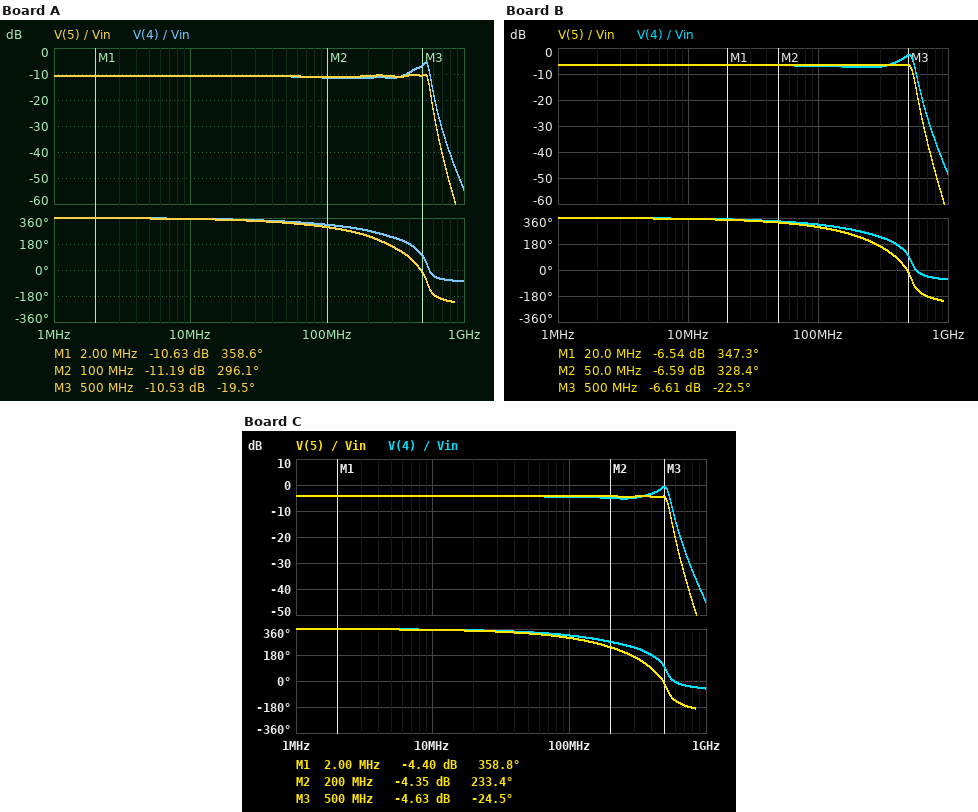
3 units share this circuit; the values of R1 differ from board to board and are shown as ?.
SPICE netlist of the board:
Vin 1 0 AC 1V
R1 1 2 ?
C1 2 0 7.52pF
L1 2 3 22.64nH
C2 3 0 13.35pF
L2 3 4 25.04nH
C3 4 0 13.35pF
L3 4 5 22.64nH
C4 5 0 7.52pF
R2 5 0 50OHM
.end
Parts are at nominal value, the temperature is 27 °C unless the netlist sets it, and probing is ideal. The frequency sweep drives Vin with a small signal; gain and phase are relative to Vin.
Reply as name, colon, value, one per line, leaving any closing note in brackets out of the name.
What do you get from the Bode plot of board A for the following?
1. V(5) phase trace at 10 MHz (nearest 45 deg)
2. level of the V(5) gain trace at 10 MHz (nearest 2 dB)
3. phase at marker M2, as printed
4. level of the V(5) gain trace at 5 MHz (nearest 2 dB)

V(5) phase trace at 10 MHz: 360 deg
level of the V(5) gain trace at 10 MHz: -10 dB
phase at marker M2, as printed: 296.1 deg
level of the V(5) gain trace at 5 MHz: -10 dB
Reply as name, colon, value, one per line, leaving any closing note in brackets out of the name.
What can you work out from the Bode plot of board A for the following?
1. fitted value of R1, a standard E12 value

fitted value of R1, a standard E12 value: 120 Ω
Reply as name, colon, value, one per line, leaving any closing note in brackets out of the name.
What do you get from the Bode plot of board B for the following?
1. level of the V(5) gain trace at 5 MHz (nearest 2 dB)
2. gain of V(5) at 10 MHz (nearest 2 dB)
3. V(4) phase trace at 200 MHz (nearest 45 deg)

level of the V(5) gain trace at 5 MHz: -6 dB
gain of V(5) at 10 MHz: -6 dB
V(4) phase trace at 200 MHz: 270 deg
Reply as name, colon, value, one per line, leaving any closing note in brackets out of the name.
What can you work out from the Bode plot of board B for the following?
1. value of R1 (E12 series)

value of R1: 56 Ω
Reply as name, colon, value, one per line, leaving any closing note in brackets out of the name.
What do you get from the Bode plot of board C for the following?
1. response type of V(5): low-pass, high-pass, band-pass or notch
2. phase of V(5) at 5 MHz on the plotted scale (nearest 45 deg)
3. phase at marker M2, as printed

response type of V(5): low-pass, high-pass, band-pass or notch: low-pass
phase of V(5) at 5 MHz on the plotted scale: 360 deg
phase at marker M2, as printed: 233.4 deg
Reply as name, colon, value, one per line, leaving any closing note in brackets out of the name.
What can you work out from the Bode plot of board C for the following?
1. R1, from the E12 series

R1, from the E12 series: 33 Ω
